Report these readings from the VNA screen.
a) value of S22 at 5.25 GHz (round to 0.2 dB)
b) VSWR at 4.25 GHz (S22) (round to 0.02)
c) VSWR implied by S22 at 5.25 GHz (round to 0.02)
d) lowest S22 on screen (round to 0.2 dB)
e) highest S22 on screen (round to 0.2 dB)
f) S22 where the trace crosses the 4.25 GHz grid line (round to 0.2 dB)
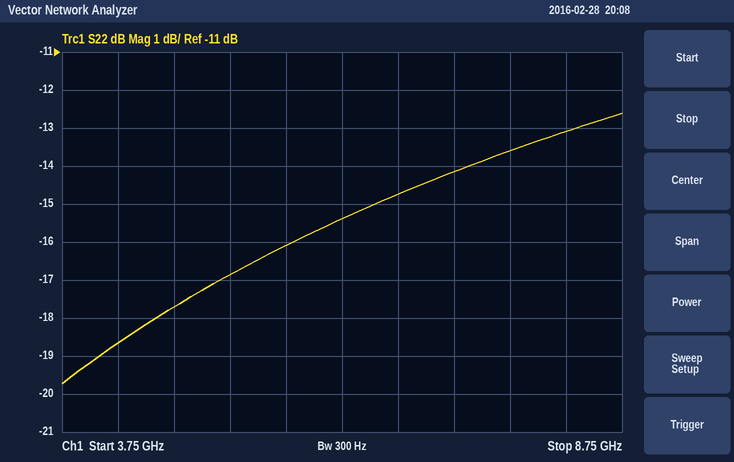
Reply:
-16.8 dB
1.26
1.34
-19.8 dB
-12.6 dB
-18.6 dB
